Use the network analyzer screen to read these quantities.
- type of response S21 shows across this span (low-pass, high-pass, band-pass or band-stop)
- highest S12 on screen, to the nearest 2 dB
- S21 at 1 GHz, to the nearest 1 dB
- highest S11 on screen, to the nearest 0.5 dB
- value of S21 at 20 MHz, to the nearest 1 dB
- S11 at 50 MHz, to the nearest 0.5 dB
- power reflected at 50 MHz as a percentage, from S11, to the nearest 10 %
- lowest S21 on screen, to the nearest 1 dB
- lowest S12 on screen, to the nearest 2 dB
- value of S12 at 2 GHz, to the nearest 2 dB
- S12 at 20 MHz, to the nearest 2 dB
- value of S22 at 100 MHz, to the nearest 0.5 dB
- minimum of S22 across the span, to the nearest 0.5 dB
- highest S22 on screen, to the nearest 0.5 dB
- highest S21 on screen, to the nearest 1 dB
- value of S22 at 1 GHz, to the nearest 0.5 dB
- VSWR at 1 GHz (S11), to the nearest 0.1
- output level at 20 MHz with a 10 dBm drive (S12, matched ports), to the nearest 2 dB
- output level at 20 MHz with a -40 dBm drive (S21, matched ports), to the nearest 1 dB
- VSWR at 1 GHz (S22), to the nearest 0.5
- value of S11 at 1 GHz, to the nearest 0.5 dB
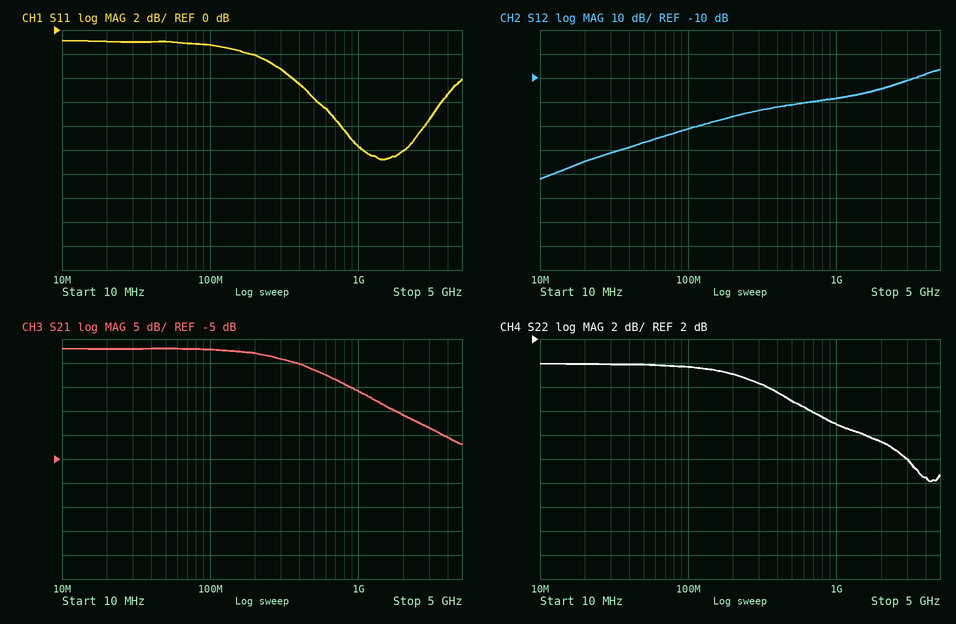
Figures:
low-pass
-6 dB
9 dB
-1.0 dB
18 dB
-1.0 dB
80 %
-2 dB
-52 dB
-14 dB
-44 dB
-0.5 dB
-10.0 dB
0.0 dB
18 dB
-5.0 dB
2.0
-34 dBm
-22 dBm
3.5
-9.5 dB
